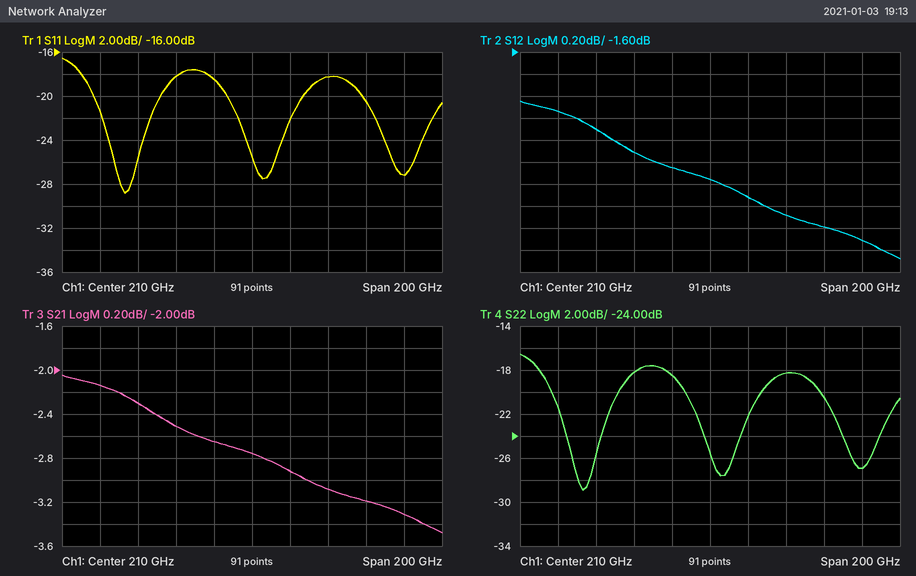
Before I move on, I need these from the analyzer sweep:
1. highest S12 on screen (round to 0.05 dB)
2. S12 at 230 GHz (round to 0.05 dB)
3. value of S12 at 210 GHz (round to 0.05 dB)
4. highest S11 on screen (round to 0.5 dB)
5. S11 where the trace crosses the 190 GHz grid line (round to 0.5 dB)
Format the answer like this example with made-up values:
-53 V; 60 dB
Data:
-2.05 dB; -2.90 dB; -2.75 dB; -16.5 dB; -18.5 dB
